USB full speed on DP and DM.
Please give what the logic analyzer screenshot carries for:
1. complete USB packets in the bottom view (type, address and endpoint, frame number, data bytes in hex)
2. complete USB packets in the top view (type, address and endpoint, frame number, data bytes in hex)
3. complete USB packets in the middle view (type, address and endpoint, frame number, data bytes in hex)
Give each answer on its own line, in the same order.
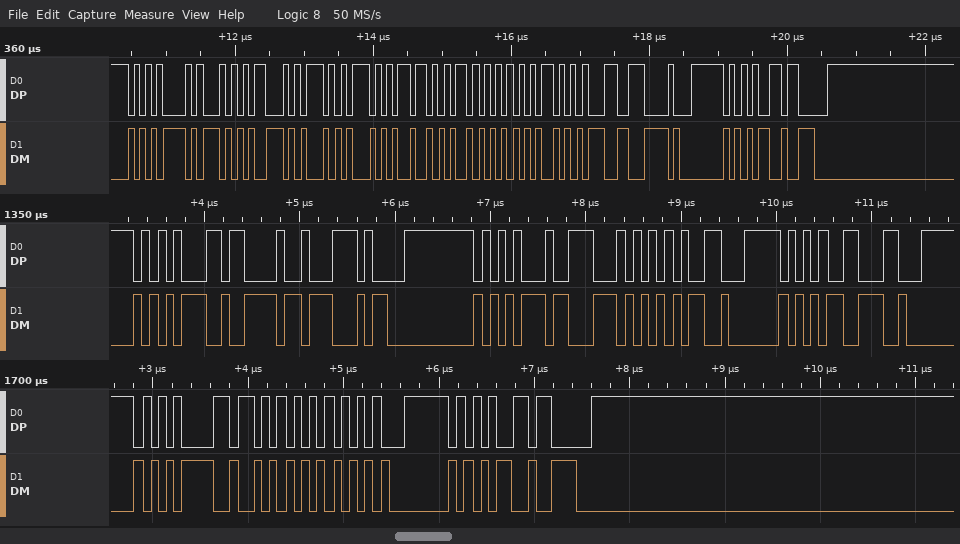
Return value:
DATA1 [ ], ACK
DATA0 [ 80 06 03 03 09 04 00 02 ], ACK
SOF 1427, IN ADDR 3 EP 0, NAK
